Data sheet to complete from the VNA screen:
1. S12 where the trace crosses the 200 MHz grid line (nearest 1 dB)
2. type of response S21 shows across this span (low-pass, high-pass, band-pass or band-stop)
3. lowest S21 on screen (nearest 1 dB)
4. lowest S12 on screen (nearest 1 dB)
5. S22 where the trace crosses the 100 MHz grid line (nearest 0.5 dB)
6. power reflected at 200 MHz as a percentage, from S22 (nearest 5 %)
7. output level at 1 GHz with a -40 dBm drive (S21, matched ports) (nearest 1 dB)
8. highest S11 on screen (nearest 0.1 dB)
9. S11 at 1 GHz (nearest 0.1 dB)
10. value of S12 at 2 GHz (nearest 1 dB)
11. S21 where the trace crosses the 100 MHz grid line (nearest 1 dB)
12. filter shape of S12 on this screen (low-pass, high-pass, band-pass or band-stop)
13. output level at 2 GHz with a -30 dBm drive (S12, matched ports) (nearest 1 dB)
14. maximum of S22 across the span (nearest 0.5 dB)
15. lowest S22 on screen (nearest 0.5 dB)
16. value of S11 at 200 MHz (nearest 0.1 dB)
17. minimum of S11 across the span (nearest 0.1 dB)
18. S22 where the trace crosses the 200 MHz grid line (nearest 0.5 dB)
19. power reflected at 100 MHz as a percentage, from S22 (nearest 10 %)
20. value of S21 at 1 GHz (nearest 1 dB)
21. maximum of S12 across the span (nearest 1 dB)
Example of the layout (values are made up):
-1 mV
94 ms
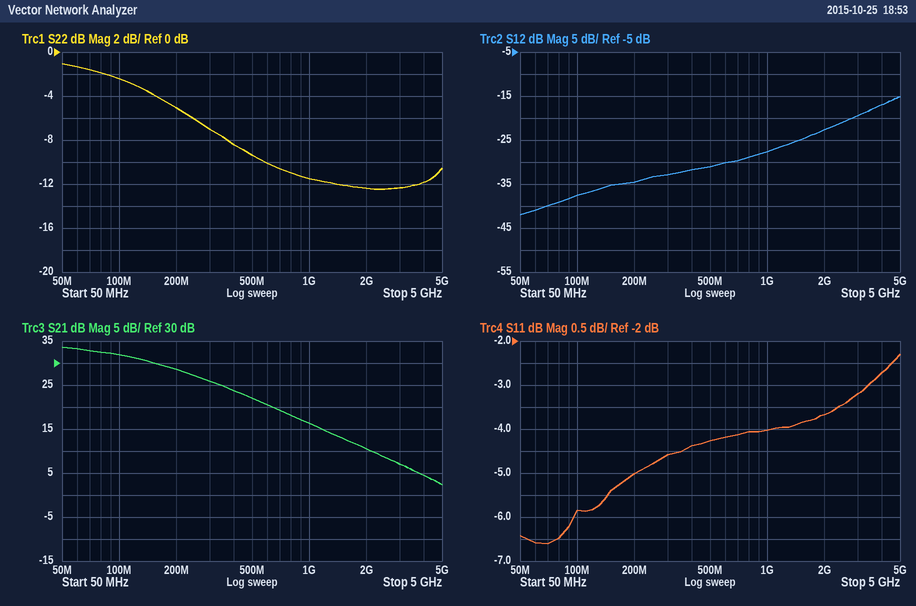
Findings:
-35 dB
low-pass
2 dB
-42 dB
-2.5 dB
30 %
-24 dBm
-2.3 dB
-4.0 dB
-23 dB
32 dB
high-pass
-53 dBm
-1.0 dB
-12.5 dB
-5.0 dB
-6.6 dB
-5.0 dB
60 %
16 dB
-15 dB
